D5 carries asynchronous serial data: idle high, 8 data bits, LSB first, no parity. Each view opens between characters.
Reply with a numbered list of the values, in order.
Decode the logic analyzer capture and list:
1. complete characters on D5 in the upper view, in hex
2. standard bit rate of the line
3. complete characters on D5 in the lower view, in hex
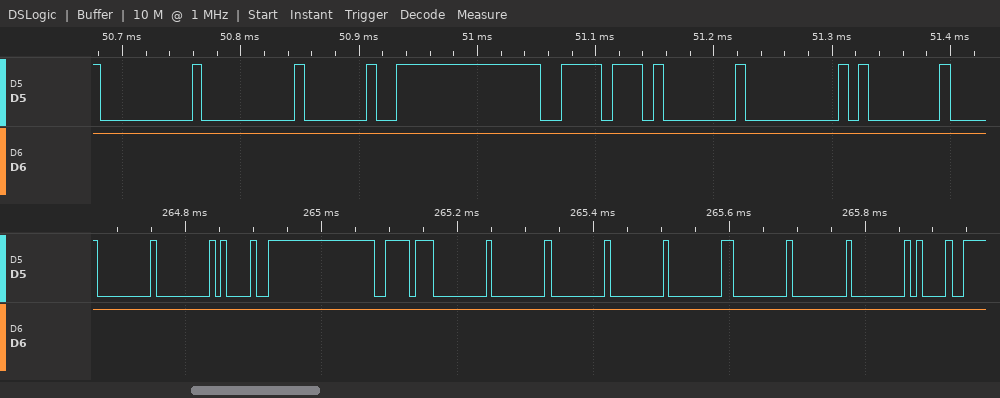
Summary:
1. 00, 00, 20, DE, 01, 00, 01
2. 115200 baud
3. 00, 00, 21, DE, 00, 00, 00, 00, 00, 00, 00, 00, 21
